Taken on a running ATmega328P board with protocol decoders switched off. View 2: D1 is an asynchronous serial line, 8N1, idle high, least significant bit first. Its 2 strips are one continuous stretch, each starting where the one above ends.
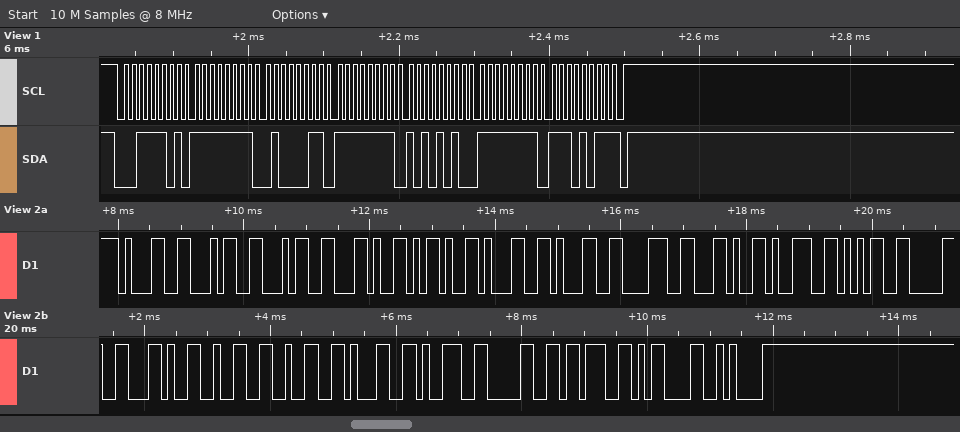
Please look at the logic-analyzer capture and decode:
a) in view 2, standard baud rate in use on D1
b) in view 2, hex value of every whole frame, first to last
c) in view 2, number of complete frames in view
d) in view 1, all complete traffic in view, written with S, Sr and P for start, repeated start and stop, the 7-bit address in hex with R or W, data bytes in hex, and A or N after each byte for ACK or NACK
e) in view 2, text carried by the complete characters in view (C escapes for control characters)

9600 baud
31 34 34 2C 2D 31 31 38 2C 39 35 30 2C 32 32 31 39 30 3B 0D 0A
21
S 1ER A FF A 43 A FF A AA A FF A EB N P
"144,-118,950,22190;\r\n"
